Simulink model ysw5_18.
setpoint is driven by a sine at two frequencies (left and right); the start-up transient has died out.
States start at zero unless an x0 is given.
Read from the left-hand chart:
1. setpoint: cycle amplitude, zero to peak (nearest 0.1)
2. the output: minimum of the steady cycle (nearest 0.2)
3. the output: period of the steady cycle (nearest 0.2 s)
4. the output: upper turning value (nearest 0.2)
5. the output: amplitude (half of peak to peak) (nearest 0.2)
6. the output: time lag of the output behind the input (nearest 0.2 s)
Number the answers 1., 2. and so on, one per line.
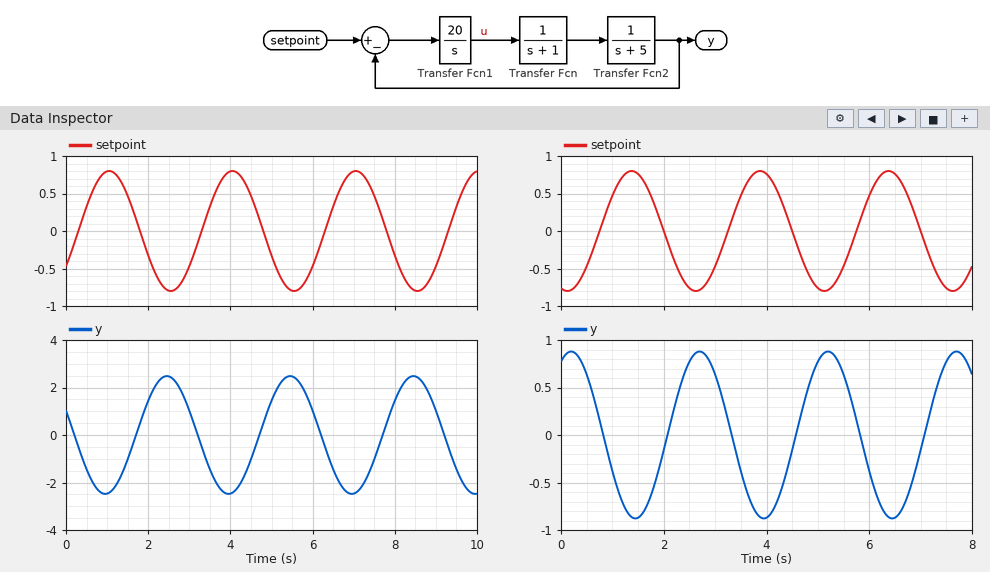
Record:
1. 0.8
2. -2.4
3. 3.0 s
4. 2.4
5. 2.4
6. 1.4 s
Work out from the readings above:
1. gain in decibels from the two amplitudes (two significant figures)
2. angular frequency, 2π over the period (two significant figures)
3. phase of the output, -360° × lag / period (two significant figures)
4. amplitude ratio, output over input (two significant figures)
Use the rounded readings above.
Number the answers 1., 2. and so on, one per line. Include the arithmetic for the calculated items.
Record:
1. 20 log10(2.4 / 0.8) = 9.5 dB
2. 2π / 3 = 2.1 rad/s
3. -360 × 1.4 / 3 = -170°
4. 2.4 / 0.8 = 3.0
